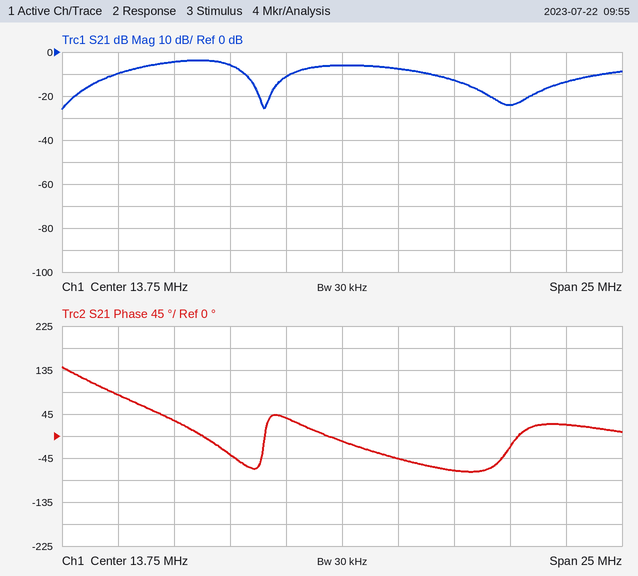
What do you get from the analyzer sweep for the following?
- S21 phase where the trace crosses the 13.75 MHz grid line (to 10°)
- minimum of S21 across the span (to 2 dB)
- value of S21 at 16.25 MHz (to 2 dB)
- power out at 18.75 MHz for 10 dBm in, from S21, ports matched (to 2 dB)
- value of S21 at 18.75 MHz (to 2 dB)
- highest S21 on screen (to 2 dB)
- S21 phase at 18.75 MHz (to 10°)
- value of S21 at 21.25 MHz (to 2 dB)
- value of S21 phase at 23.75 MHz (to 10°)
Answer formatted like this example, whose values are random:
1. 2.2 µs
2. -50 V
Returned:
1. -10°
2. -26 dB
3. -8 dB
4. -2 dBm
5. -12 dB
6. -4 dB
7. -70°
8. -24 dB
9. 20°
